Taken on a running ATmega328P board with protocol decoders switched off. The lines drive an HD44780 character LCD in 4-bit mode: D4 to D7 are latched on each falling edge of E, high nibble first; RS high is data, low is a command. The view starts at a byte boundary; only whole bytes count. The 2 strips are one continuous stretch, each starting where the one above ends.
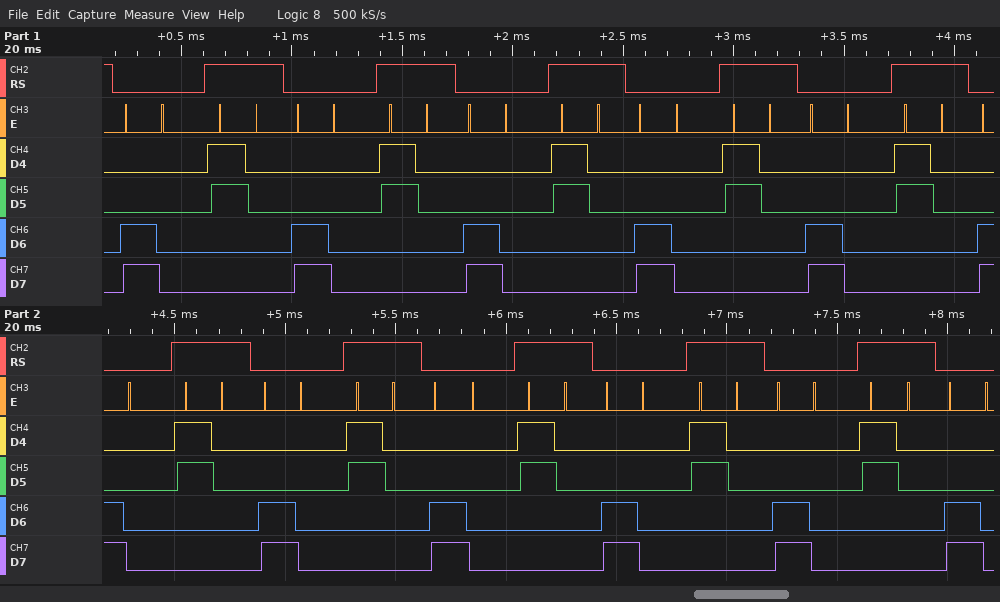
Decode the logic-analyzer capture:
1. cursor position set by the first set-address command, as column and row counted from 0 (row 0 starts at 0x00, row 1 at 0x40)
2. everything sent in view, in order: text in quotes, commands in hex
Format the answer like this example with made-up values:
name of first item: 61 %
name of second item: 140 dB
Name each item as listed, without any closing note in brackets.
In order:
cursor position set by the first set-address command, as column and row counted from 0: column 0, row 1
everything sent in view, in order: text in quotes, commands in hex: 0xC0 "0" 0xC0 "0" 0xC0 "0" 0xC0 "0" 0xC0 "0" 0xC0 "0" 0xC0 "0" 0xC0 "0" 0xC0 "0" 0xC0 "0" 0xC0
